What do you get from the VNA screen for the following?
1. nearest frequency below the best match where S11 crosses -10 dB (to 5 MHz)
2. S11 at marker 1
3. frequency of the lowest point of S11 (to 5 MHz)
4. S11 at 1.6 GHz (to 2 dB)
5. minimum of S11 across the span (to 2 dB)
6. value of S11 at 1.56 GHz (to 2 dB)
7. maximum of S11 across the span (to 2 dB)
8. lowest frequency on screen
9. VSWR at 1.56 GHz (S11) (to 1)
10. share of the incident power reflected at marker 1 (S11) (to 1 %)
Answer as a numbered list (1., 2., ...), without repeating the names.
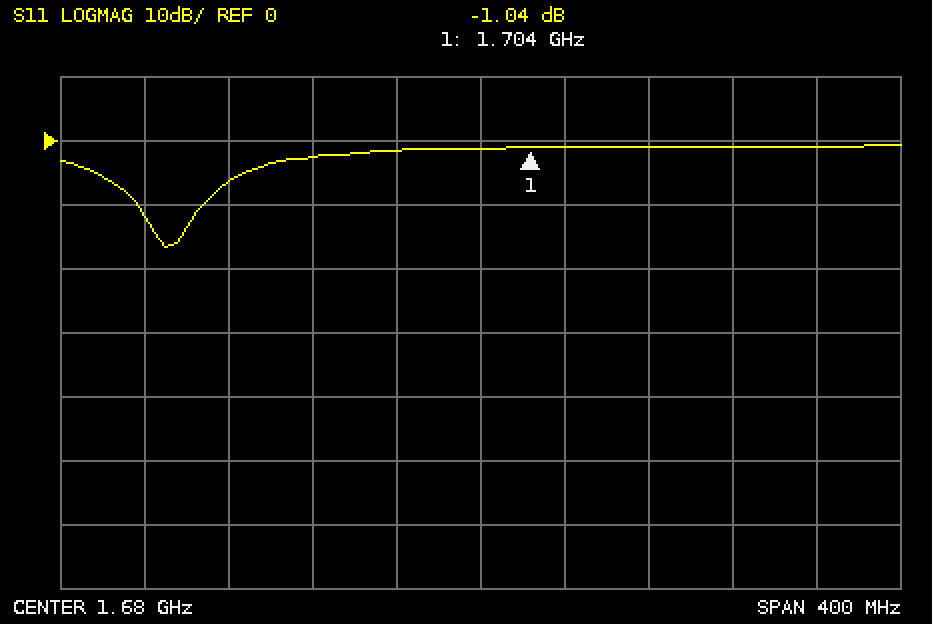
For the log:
1. 1.515 GHz
2. -1.04 dB
3. 1.530 GHz
4. -2 dB
5. -16 dB
6. -6 dB
7. 0 dB
8. 1.48 GHz
9. 3
10. 79 %
